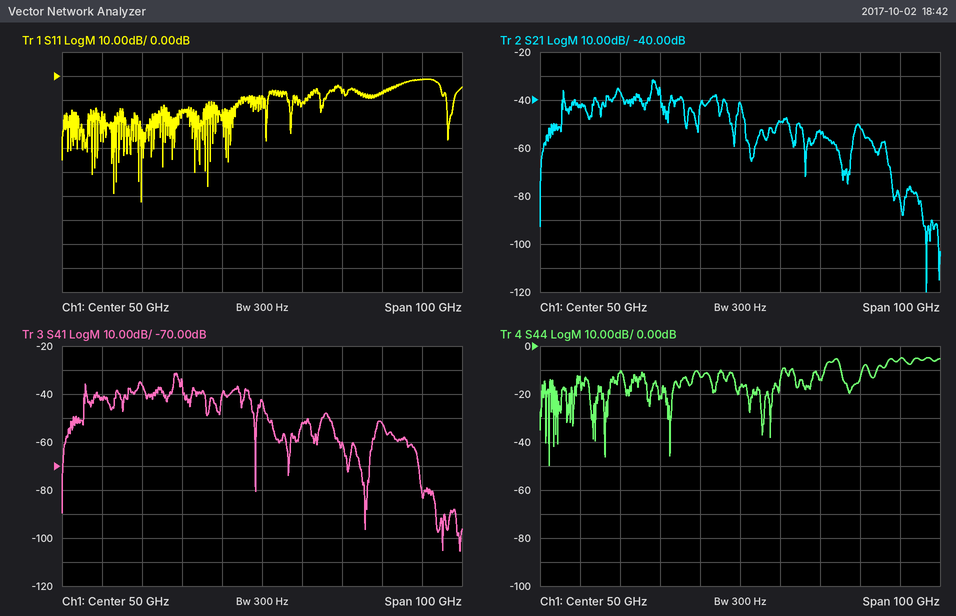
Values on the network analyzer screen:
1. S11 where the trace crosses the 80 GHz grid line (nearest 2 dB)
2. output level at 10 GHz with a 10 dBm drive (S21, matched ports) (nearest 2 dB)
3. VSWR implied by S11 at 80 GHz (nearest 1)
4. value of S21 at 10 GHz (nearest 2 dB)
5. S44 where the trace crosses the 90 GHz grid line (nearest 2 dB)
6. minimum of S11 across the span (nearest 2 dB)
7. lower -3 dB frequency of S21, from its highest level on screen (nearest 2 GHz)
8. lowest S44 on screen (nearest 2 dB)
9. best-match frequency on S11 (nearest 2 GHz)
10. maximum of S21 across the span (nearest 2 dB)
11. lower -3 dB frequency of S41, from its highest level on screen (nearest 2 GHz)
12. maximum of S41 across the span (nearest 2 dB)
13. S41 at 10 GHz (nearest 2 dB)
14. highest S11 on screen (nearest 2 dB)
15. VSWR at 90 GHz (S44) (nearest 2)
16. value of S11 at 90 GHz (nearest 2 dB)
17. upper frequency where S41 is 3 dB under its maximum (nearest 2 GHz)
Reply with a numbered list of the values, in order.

1. -6 dB
2. -32 dBm
3. 3
4. -42 dB
5. -6 dB
6. -52 dB
7. 28 GHz
8. -50 dB
9. 20 GHz
10. -32 dB
11. 28 GHz
12. -32 dB
13. -42 dB
14. -2 dB
15. 4
16. -2 dB
17. 30 GHz
